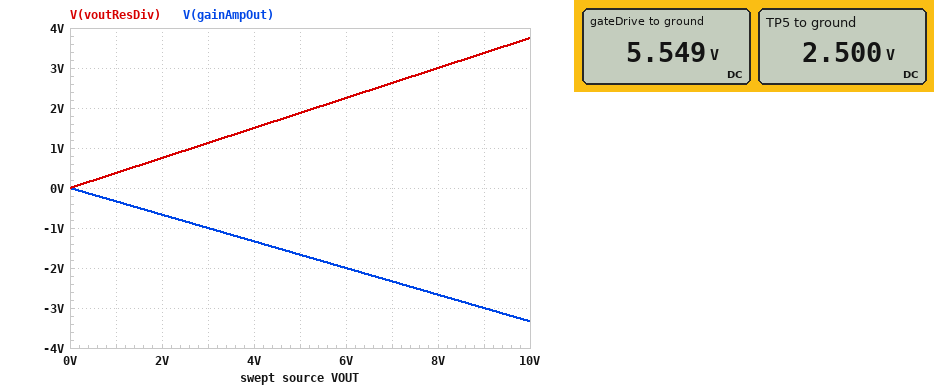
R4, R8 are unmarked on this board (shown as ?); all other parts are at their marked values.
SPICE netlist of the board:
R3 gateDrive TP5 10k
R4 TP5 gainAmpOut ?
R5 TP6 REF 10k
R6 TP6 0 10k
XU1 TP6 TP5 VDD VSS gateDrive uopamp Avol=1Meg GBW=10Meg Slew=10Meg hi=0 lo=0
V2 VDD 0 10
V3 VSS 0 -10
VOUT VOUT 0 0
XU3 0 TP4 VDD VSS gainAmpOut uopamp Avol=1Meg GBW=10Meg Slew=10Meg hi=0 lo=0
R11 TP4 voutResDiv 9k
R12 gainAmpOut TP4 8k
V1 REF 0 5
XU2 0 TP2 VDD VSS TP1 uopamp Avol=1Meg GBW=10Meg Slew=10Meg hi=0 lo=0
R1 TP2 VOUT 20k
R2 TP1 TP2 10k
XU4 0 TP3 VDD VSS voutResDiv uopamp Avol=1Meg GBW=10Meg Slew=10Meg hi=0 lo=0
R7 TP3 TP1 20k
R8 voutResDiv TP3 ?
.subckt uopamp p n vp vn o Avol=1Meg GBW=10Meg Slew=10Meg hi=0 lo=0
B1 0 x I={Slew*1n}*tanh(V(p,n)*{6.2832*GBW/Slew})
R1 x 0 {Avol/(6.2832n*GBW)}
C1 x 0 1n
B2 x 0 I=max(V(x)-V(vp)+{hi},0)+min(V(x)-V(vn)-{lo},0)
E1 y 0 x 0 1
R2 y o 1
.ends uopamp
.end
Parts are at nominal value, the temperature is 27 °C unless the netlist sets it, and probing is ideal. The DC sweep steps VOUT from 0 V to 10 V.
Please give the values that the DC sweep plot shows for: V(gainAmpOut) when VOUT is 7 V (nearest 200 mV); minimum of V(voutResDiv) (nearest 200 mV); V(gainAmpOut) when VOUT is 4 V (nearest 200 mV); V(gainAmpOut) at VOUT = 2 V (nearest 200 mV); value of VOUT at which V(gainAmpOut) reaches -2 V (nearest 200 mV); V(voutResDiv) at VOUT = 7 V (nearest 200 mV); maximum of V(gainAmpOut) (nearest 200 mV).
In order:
-2.4 V
0 V
-1.4 V
-600 mV
6.0 V
2.6 V
0 V
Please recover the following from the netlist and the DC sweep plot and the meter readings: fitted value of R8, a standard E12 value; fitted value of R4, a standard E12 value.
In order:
15 kΩ
8.2 kΩ
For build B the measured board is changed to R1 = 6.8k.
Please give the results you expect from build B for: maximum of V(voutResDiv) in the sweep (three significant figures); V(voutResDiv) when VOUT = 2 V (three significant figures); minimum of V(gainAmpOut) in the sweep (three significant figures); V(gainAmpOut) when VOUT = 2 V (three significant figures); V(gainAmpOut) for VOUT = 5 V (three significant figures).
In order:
7.51 V
2.21 V
-6.67 V
-1.96 V
-4.90 V
